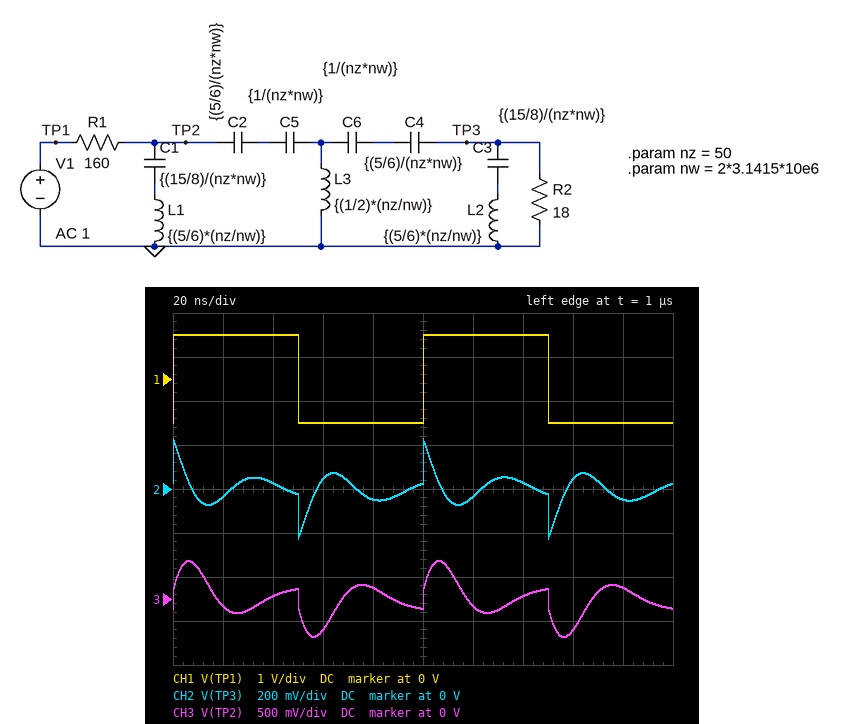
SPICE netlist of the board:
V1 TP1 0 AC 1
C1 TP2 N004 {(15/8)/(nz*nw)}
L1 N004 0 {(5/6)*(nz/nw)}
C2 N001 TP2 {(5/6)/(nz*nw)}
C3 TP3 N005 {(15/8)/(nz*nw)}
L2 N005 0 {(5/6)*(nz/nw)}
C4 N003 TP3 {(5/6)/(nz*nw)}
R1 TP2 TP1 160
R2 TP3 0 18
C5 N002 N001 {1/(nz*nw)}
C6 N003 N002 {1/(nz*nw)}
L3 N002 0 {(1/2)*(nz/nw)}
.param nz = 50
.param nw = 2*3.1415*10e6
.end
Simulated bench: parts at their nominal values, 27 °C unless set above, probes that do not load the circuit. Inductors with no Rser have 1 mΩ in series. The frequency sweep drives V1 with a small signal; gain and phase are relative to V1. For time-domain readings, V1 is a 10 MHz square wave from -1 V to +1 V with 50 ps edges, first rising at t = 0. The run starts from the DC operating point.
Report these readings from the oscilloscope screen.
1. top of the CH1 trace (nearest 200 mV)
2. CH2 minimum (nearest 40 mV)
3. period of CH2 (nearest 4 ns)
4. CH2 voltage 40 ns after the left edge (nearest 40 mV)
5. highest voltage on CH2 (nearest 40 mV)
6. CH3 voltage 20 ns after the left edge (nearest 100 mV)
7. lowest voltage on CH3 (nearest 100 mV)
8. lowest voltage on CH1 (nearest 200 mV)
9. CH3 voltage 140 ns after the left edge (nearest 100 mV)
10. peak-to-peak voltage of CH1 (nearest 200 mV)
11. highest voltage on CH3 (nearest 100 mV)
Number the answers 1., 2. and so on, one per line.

1. 1.0 V
2. -240 mV
3. 100 ns
4. 40 mV
5. 240 mV
6. -100 mV
7. -400 mV
8. -1.0 V
9. 0 V
10. 2.0 V
11. 400 mV
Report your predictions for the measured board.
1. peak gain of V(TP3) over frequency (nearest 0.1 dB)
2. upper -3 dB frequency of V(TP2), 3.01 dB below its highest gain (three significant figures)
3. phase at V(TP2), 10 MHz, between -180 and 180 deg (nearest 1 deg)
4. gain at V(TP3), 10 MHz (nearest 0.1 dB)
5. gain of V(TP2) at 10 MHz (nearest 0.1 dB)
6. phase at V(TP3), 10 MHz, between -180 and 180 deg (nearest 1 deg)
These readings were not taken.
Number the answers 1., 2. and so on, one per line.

1. -15.5 dB
2. 1.31 MHz
3. 83 deg
4. -44.9 dB
5. -18.7 dB
6. 37 deg
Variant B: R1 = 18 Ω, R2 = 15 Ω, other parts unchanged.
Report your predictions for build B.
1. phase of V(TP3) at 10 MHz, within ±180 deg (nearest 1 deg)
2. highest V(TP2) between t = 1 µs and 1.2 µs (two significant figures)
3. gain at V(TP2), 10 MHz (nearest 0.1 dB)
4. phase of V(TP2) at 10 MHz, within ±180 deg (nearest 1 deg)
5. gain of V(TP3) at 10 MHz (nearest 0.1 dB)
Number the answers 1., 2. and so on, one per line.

1. -7 deg
2. 1.4 V
3. -2.9 dB
4. 44 deg
5. -30.0 dB
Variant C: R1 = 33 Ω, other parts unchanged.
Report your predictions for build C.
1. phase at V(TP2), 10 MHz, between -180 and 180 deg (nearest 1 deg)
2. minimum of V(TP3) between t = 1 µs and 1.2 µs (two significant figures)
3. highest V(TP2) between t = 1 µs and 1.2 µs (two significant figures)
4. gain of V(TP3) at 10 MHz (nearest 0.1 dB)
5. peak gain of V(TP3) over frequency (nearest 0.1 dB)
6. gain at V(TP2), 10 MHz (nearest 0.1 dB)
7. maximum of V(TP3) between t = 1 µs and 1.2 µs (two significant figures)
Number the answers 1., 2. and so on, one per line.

1. 60 deg
2. -720 mV
3. 1.2 V
4. -32.4 dB
5. -8.9 dB
6. -6.2 dB
7. 720 mV
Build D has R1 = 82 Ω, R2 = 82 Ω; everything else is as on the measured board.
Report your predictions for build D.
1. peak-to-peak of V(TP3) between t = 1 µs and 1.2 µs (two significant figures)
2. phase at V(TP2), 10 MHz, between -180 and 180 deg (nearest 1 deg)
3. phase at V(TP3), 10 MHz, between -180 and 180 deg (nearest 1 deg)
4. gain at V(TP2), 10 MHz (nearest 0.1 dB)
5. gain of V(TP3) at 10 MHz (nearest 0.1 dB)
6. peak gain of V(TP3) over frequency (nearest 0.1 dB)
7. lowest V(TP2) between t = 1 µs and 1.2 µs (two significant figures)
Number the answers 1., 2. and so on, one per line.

1. 2.1 V
2. 77 deg
3. 64 deg
4. -13.1 dB
5. -36.3 dB
6. -6.0 dB
7. -900 mV
